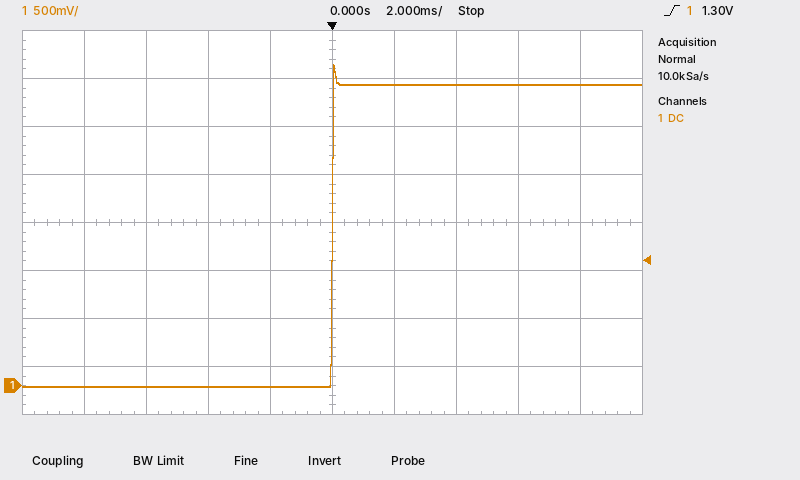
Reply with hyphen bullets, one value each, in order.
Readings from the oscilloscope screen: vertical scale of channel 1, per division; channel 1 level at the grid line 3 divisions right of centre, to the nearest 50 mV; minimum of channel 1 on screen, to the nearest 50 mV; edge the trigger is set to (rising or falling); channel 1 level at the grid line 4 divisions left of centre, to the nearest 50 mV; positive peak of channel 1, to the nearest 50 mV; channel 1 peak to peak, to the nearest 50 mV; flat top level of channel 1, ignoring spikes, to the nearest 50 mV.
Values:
- 500 mV
- 3.15 V
- 0 mV
- rising
- 0 mV
- 3.35 V
- 3.35 V
- 3.15 V
